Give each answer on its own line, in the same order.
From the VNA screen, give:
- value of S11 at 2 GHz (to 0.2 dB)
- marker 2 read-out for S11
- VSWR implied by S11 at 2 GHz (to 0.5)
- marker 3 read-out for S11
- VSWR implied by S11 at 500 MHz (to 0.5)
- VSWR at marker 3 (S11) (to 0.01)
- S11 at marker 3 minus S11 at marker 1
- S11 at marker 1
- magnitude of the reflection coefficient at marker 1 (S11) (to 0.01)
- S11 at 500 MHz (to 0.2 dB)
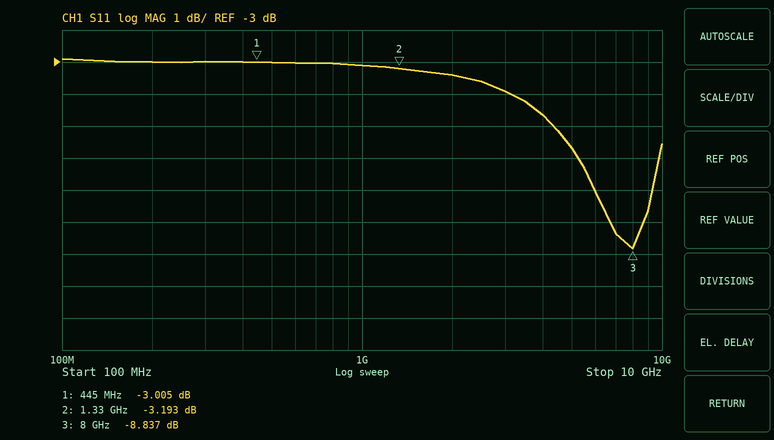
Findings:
-3.4 dB
-3.193 dB
5.0
-8.837 dB
6.0
2.13
-5.832 dB
-3.005 dB
0.71
-3.0 dB
